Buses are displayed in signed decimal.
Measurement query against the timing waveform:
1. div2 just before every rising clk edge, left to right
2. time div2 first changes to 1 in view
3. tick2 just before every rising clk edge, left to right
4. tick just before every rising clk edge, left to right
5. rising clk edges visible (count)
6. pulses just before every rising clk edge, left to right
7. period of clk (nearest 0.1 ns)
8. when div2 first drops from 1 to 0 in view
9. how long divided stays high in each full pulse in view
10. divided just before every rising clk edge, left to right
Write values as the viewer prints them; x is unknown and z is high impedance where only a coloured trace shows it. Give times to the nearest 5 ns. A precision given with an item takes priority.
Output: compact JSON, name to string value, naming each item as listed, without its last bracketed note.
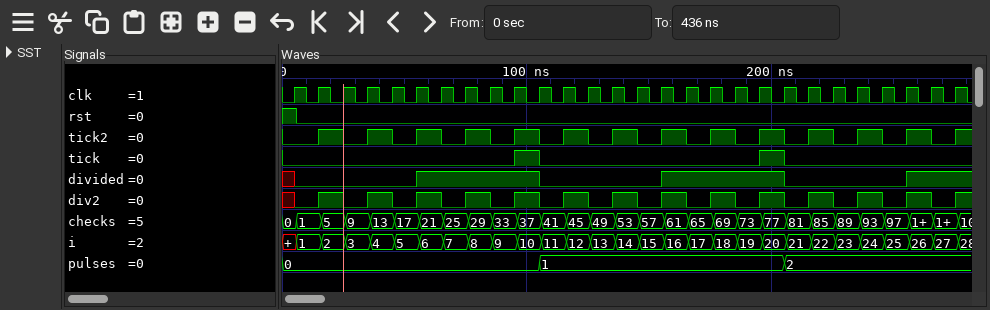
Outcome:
{"div2 just before every rising clk edge, left to right": "x 0 1 0 1 0 1 0 1 0 1 0 1 0 1 0 1 0 1 0 1 0 1 0 1 0 1 0", "time div2 first changes to 1 in view": "15 ns", "tick2 just before every rising clk edge, left to right": "0 0 1 0 1 0 1 0 1 0 1 0 1 0 1 0 1 0 1 0 1 0 1 0 1 0 1 0", "tick just before every rising clk edge, left to right": "0 0 0 0 0 0 0 0 0 0 1 0 0 0 0 0 0 0 0 0 1 0 0 0 0 0 0 0", "rising clk edges visible": "28", "pulses just before every rising clk edge, left to right": "0, 0, 0, 0, 0, 0, 0, 0, 0, 0, 0, 1, 1, 1, 1, 1, 1, 1, 1, 1, 1, 2, 2, 2, 2, 2, 2, 2", "period of clk": "10 ns", "when div2 first drops from 1 to 0 in view": "25 ns", "how long divided stays high in each full pulse in view": "50 ns, 50 ns", "divided just before every rising clk edge, left to right": "x 0 0 0 0 0 1 1 1 1 1 0 0 0 0 0 1 1 1 1 1 0 0 0 0 0 1 1"}
